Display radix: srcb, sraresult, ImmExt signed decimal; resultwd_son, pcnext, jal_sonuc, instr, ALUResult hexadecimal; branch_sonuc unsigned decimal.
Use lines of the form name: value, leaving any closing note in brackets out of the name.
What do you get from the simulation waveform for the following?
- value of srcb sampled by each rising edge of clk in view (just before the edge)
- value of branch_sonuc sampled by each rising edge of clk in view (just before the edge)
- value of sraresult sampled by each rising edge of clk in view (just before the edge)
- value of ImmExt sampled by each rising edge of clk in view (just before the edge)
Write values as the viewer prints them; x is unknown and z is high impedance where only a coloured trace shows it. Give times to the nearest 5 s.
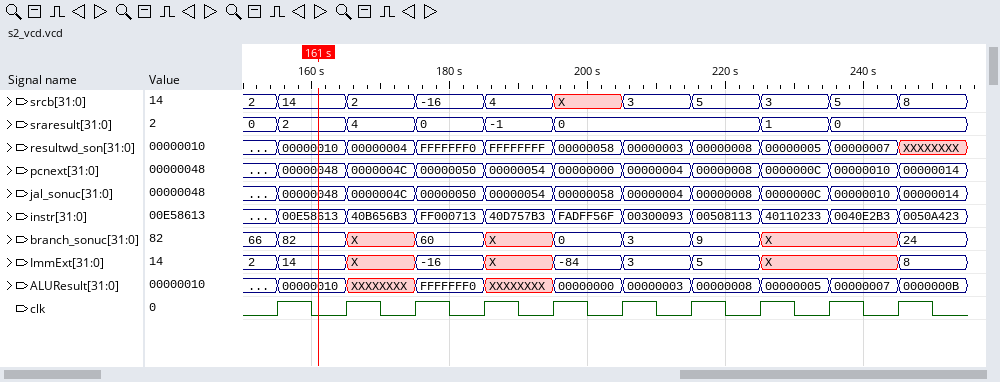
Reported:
value of srcb sampled by each rising edge of clk in view: 2, 14, 2, -16, 4, X, 3, 5, 3, 5
value of branch_sonuc sampled by each rising edge of clk in view: 66, 82, X, 60, X, 0, 3, 9, X, X
value of sraresult sampled by each rising edge of clk in view: 0, 2, 4, 0, -1, 0, 0, 0, 1, 0
value of ImmExt sampled by each rising edge of clk in view: 2, 14, X, -16, X, -84, 3, 5, X, X
